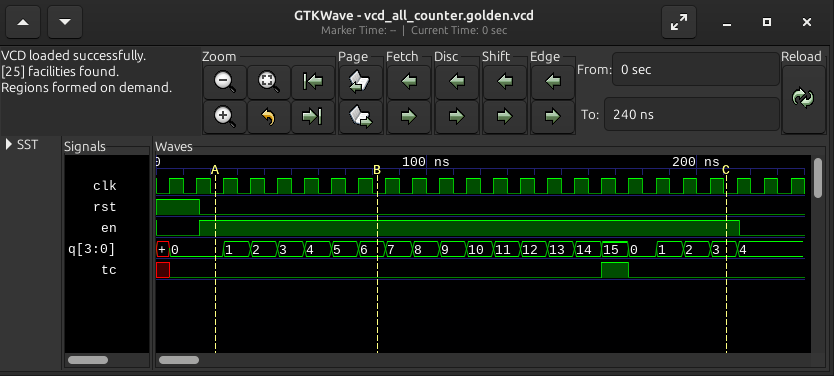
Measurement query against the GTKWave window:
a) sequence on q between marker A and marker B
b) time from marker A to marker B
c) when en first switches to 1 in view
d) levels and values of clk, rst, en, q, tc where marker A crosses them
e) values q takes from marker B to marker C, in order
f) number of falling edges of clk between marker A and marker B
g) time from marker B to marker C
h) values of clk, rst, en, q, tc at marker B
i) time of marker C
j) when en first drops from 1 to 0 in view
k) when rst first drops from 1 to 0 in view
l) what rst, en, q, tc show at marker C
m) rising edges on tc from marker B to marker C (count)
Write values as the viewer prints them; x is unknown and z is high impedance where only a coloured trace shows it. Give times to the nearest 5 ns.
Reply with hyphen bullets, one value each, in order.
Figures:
- 0, 1, 2, 3, 4, 5, 6
- 60 ns
- 15 ns
- clk=0, rst=0, en=1, q=0, tc=0
- 6, 7, 8, 9, 10, 11, 12, 13, 14, 15, 0, 1, 2, 3
- 6
- 130 ns
- clk=0, rst=0, en=1, q=6, tc=0
- 210 ns
- 215 ns
- 15 ns
- rst=0, en=1, q=3, tc=0
- 1
